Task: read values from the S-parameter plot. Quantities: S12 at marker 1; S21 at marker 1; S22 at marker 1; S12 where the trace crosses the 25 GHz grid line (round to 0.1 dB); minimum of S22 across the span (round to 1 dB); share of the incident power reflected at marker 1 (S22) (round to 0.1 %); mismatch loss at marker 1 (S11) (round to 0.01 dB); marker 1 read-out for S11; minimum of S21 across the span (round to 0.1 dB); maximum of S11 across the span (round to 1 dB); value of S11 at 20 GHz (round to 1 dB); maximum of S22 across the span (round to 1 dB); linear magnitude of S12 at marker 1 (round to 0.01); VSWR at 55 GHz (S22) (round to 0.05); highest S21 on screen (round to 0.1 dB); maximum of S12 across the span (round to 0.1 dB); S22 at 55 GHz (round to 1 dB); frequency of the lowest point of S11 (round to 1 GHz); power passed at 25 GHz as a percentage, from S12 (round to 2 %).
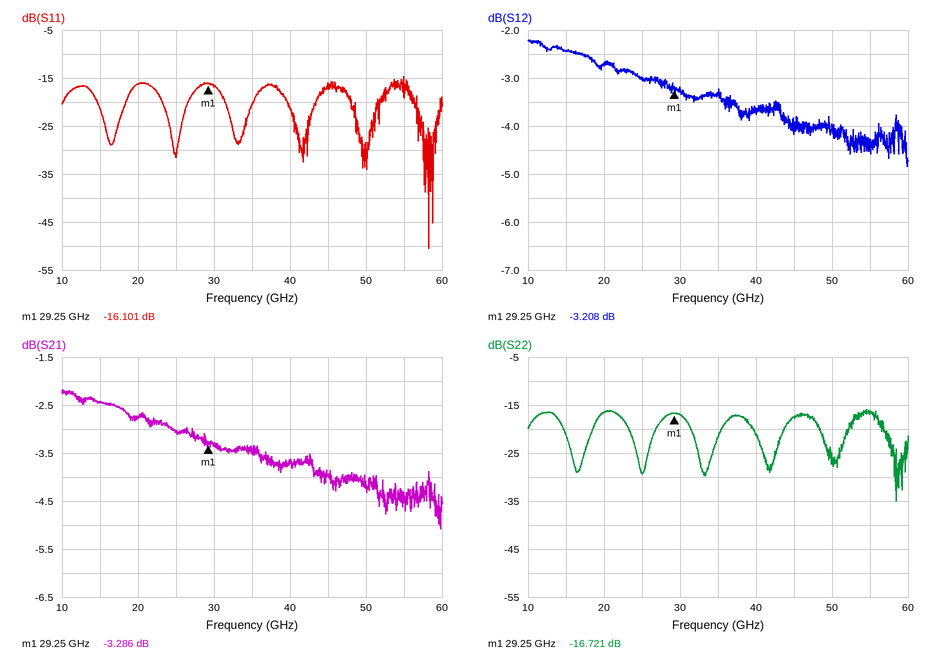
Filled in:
-3.208 dB
-3.286 dB
-16.721 dB
-3.0 dB
-35 dB
2.1 %
0.11 dB
-16.101 dB
-5.1 dB
-15 dB
-16 dB
-16 dB
0.69
1.35
-2.2 dB
-2.2 dB
-17 dB
58 GHz
50 %
